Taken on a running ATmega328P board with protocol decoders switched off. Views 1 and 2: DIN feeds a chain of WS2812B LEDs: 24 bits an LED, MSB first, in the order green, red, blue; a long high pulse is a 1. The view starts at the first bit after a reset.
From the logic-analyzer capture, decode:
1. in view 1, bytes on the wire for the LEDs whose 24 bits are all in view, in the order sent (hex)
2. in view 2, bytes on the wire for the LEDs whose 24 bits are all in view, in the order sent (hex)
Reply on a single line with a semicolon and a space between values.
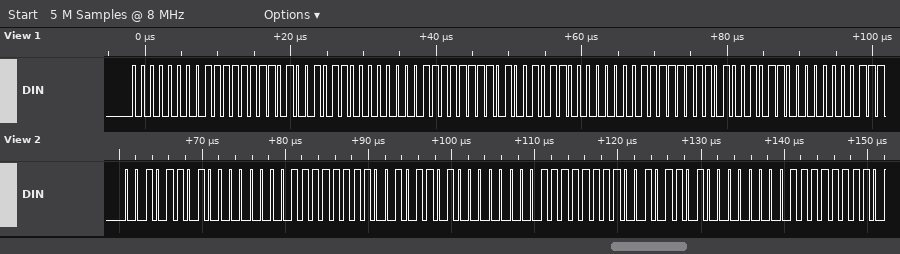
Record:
00 FF 4B 00 FF 4B 00 FF 4B; 2D 00 FF 2D 00 FF 2D 00 FF
